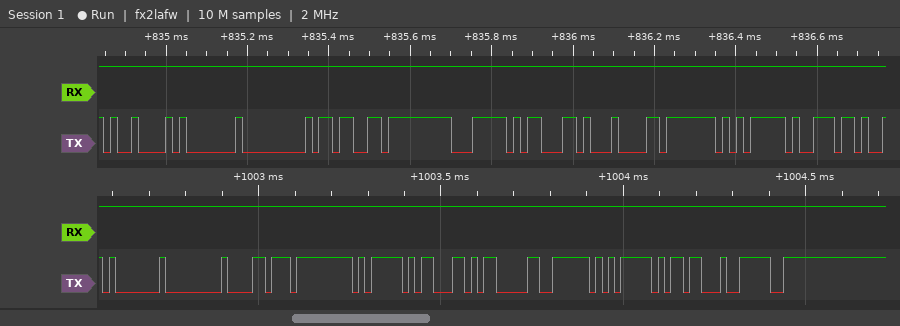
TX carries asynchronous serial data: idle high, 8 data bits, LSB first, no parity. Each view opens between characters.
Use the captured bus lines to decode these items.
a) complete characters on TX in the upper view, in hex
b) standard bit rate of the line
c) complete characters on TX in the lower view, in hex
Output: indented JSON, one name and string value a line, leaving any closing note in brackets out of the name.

{
  "complete characters on TX in the upper view, in hex": "09, 01, 00, 9B, FF, 7C, 63, 84, 7F, 7D, 6E",
  "standard bit rate of the line": "57600 baud",
  "complete characters on TX in the lower view, in hex": "01, 00, D8, FF, 7D, 63, 83, 7E, 7D, 1B, 3E"
}
